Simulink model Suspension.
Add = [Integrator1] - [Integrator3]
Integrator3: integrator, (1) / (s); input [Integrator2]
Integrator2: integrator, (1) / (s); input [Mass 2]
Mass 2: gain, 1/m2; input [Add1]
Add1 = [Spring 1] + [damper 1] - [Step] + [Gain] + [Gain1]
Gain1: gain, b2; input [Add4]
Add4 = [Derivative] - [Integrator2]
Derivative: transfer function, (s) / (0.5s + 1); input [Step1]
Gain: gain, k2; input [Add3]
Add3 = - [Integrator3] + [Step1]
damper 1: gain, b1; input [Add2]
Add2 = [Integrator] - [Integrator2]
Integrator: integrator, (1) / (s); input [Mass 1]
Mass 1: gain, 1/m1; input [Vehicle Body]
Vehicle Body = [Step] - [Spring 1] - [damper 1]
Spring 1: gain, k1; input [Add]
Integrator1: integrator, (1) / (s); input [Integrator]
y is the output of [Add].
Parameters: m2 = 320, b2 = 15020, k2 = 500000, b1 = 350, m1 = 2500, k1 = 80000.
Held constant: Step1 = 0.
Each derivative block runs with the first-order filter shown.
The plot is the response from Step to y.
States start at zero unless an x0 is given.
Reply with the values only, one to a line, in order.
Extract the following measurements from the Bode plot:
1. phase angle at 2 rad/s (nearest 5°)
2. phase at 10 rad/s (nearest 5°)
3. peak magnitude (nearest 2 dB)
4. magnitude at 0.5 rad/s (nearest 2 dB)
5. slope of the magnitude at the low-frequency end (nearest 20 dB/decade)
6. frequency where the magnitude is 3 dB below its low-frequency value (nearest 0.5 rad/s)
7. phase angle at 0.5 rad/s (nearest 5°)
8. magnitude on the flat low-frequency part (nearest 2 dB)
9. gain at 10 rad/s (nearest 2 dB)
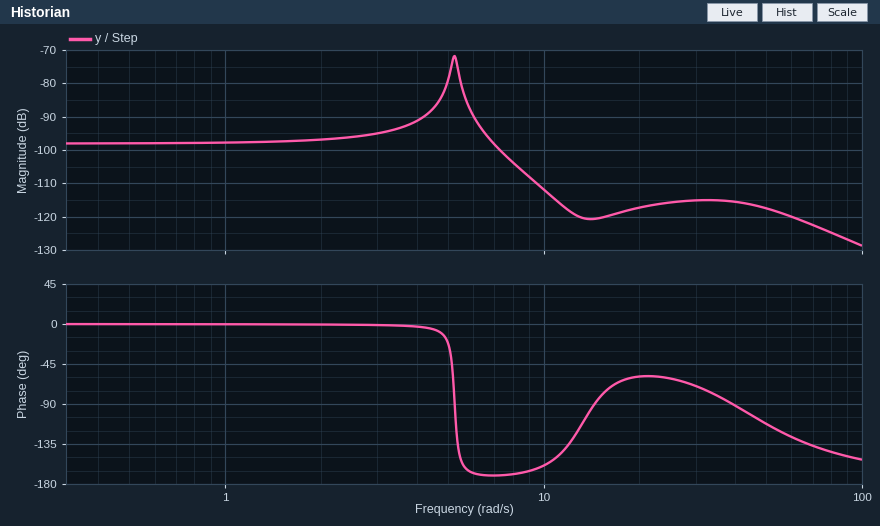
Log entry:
0°
-160°
-72 dB
-98 dB
0 dB/decade
7.5 rad/s
0°
-98 dB
-112 dB
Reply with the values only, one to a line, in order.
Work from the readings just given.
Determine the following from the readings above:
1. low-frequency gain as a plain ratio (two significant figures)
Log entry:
0.000013
